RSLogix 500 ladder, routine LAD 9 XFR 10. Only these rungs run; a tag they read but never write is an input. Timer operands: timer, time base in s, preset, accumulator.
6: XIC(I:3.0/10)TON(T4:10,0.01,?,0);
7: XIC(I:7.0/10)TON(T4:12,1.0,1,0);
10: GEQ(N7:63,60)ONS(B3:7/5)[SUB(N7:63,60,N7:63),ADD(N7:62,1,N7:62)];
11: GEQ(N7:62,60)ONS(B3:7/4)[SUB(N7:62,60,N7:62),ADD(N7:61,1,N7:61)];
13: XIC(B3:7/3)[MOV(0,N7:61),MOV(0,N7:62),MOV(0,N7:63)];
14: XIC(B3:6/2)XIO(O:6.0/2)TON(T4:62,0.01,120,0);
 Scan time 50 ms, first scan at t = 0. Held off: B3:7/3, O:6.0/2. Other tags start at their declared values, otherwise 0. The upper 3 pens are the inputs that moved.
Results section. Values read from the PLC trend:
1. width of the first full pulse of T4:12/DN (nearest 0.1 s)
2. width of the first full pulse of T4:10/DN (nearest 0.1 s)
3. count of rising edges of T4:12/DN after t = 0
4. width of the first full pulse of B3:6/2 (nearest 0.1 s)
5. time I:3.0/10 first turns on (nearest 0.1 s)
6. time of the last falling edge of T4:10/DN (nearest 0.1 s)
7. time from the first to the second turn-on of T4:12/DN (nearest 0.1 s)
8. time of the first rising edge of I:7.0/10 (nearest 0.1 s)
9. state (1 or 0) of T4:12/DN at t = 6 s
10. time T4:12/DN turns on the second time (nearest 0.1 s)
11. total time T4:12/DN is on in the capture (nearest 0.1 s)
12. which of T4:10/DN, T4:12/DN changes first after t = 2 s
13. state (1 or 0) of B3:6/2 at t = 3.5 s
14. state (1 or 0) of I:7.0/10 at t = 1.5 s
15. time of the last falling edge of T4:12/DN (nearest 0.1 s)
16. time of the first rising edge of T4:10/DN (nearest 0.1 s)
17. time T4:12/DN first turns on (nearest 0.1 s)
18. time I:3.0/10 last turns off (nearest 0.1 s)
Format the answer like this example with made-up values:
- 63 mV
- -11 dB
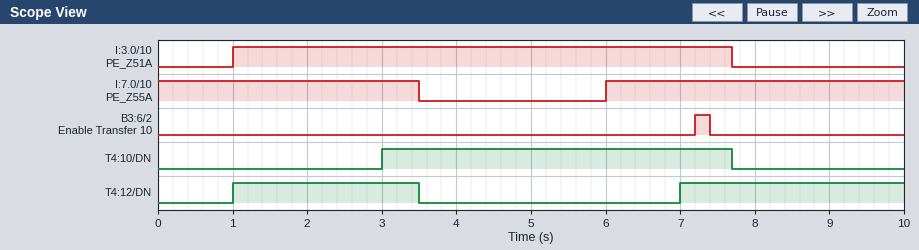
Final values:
- 2.5 s
- 4.7 s
- 2
- 0.2 s
- 1.0 s
- 7.7 s
- 6.0 s
- 6.0 s
- 0
- 7.0 s
- 5.5 s
- T4:10/DN
- 0
- 1
- 3.5 s
- 3.0 s
- 1.0 s
- 7.7 s
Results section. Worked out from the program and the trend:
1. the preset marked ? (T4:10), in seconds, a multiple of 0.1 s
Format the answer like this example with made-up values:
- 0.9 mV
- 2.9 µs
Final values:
- 2.0 s
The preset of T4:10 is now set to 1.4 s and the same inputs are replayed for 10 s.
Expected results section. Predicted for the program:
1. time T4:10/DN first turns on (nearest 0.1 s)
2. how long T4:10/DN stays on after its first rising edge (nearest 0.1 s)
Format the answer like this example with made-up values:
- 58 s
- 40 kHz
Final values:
- 2.4 s
- 5.3 s
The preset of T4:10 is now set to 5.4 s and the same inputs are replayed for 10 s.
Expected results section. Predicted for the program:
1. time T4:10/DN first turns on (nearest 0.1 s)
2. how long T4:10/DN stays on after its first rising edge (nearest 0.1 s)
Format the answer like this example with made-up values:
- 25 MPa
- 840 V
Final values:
- 6.4 s
- 1.3 s
